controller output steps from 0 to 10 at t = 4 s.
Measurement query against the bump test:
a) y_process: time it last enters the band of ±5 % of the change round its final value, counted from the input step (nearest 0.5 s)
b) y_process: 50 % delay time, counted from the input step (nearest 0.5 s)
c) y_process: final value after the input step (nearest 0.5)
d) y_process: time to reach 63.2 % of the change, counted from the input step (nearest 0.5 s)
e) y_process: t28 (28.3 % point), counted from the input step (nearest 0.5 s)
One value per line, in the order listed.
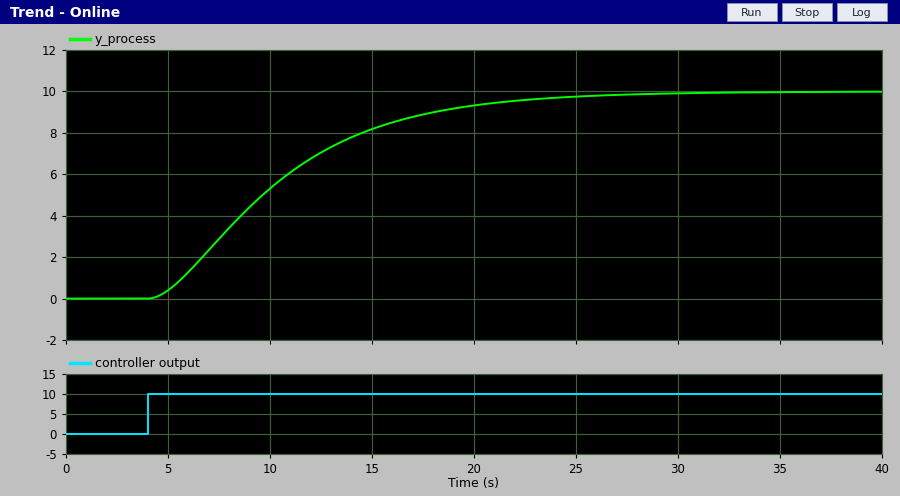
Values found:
17.5 s
5.5 s
10.0
7.5 s
3.5 s
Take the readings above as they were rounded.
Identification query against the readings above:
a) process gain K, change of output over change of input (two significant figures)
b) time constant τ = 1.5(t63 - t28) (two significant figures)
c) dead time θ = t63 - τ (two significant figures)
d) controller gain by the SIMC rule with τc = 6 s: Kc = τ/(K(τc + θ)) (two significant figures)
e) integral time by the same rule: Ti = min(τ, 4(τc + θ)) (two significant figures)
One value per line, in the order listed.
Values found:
1.0
6.0 s
1.5 s
0.80
6.0 s
